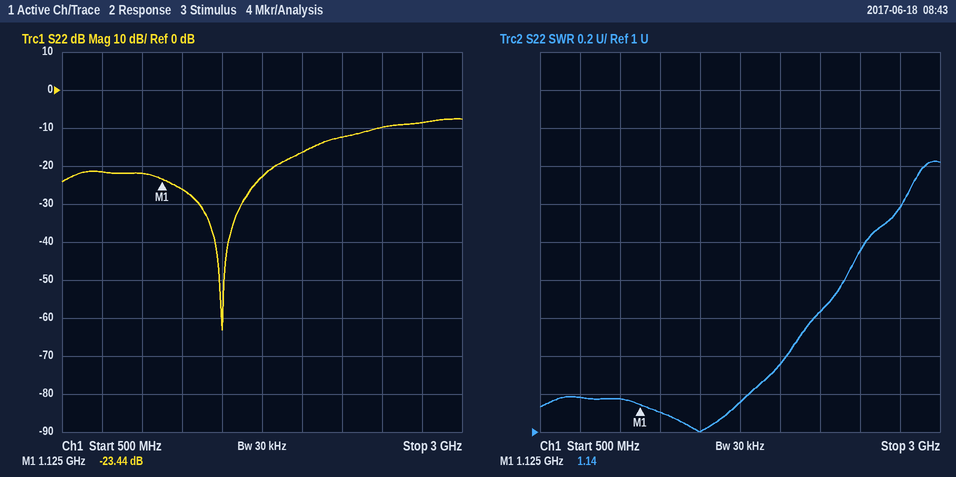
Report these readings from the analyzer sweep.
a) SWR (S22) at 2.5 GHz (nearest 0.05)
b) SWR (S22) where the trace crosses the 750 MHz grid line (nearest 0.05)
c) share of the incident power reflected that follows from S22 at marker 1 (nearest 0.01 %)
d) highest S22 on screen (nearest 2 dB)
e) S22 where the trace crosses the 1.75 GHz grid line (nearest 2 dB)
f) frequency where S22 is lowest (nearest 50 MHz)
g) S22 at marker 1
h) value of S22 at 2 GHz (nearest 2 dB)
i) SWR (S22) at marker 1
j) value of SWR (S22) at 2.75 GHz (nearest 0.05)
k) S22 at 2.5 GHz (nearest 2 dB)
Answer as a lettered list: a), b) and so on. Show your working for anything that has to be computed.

a) 1.95
b) 1.20
c) 10^(-23.44/10) ≈ 0.45 %
d) -8 dB
e) -22 dB
f) 1.50 GHz
g) -23.44 dB
h) -16 dB
i) 1.14
j) 2.20
k) -10 dB
